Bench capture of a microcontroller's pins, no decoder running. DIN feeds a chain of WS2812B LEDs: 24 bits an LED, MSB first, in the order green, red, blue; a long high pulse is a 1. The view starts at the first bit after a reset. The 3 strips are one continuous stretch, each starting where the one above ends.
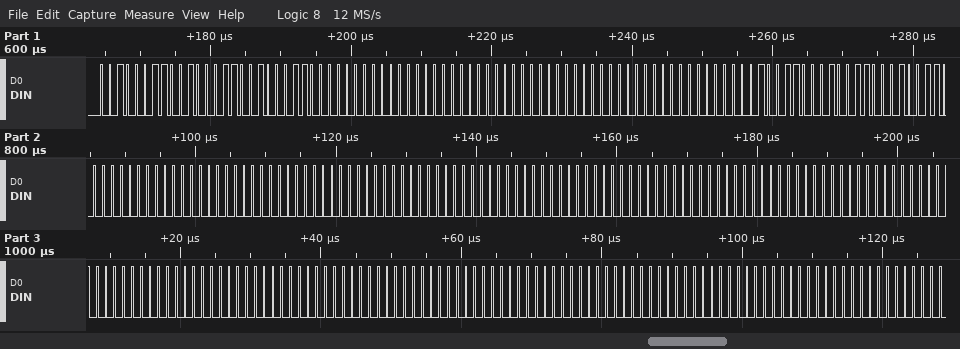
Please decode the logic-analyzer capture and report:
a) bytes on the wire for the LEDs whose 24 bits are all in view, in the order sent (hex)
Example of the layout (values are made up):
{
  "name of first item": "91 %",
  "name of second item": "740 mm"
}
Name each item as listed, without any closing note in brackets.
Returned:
{
  "bytes on the wire for the LEDs whose 24 bits are all in view, in the order sent": "23 23 23 00 00 00 00 00 00 13 13 13 00 00 00 00 00 00 00 00 00 00 00 00 00 00 00 00 00 00 00 00 00 00 00 00"
}
